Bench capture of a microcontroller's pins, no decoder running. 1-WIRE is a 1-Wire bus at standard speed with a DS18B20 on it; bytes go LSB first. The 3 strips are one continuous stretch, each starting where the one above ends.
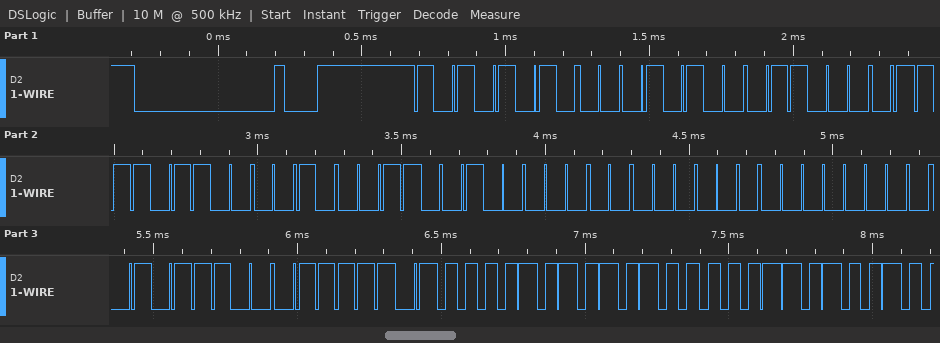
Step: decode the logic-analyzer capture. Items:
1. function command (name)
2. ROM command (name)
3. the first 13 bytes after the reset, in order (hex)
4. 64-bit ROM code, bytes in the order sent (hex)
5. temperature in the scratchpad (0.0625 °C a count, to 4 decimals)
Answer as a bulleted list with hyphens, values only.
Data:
- Read Scratchpad
- Match ROM
- 55 28 86 37 C4 04 00 00 3A BE 50 05 4B
- 28 86 37 C4 04 00 00 3A
- 85.0000 °C
